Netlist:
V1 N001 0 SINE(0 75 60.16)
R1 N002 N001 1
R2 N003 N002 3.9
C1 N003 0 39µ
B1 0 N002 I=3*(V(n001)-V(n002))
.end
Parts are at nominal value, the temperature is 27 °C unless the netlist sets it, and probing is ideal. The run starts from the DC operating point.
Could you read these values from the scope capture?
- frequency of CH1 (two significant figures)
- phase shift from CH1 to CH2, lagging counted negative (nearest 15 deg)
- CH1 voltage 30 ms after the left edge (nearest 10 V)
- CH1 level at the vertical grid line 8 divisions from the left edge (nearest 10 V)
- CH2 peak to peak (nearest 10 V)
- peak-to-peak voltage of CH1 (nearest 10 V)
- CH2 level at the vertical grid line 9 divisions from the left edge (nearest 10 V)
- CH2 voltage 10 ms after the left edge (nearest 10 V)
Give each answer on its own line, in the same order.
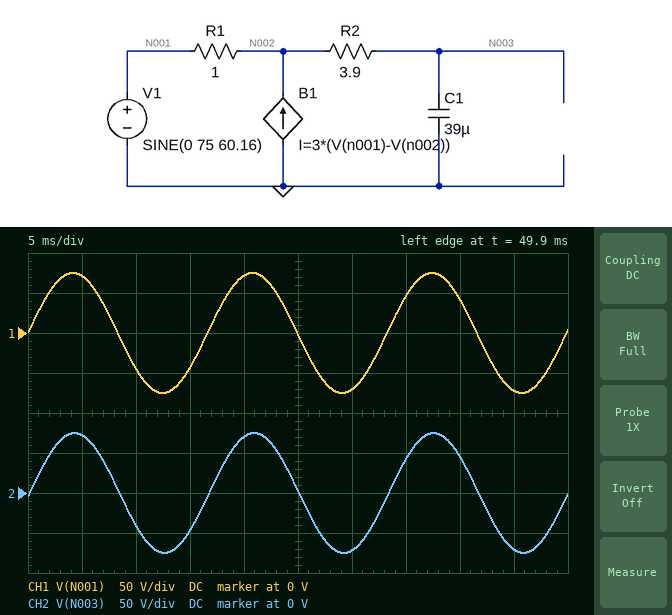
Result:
60 Hz
0 deg
-70 V
40 V
150 V
150 V
-70 V
-40 V
